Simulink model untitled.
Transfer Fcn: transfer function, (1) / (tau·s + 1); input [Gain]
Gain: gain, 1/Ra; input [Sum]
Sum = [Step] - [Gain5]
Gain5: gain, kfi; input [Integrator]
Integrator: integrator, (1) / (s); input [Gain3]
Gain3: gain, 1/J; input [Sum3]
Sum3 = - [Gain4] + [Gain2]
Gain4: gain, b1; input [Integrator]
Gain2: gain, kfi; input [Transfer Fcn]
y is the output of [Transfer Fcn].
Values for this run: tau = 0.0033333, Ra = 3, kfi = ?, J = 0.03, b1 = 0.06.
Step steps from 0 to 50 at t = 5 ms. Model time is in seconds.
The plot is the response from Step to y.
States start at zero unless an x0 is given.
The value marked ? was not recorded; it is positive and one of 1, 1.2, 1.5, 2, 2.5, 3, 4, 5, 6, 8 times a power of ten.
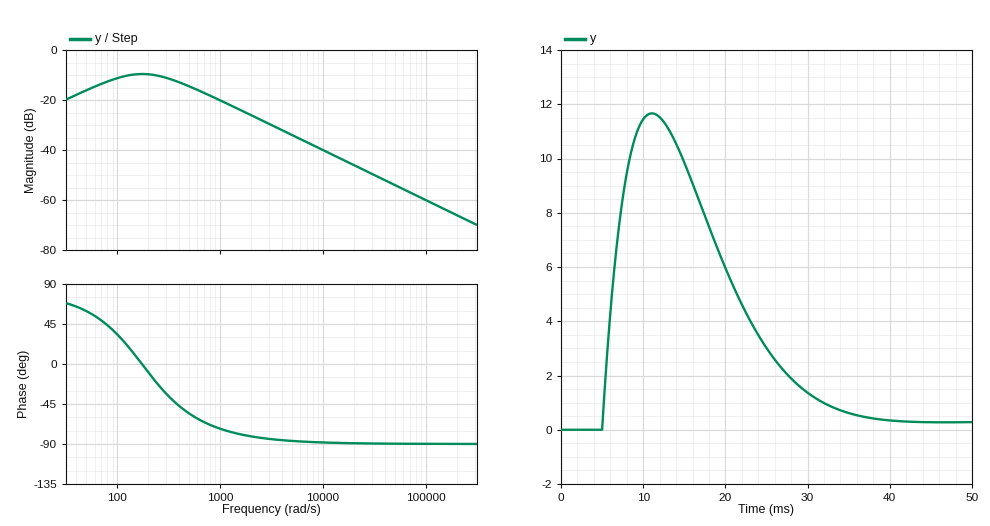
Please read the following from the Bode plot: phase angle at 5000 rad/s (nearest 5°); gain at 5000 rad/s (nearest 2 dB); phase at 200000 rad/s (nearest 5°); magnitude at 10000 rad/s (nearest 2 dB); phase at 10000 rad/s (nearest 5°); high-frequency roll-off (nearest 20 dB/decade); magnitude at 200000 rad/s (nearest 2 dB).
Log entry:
-85°
-34 dB
-90°
-40 dB
-90°
-20 dB/decade
-66 dB
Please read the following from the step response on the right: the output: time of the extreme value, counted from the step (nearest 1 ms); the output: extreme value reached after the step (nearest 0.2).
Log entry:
6 ms
11.6
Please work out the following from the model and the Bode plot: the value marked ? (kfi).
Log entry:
3
